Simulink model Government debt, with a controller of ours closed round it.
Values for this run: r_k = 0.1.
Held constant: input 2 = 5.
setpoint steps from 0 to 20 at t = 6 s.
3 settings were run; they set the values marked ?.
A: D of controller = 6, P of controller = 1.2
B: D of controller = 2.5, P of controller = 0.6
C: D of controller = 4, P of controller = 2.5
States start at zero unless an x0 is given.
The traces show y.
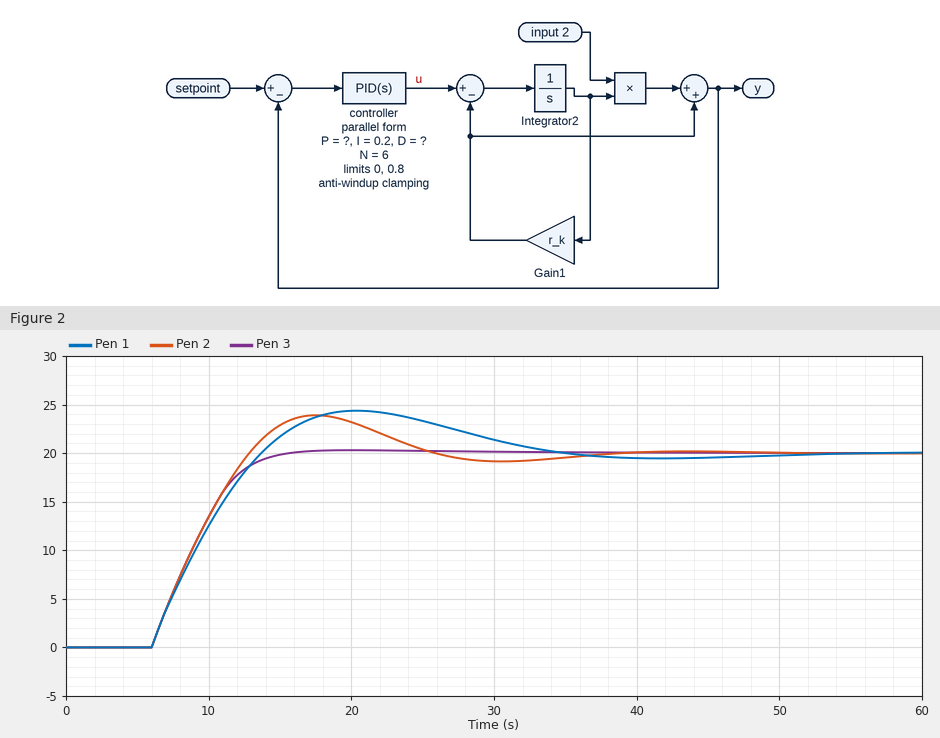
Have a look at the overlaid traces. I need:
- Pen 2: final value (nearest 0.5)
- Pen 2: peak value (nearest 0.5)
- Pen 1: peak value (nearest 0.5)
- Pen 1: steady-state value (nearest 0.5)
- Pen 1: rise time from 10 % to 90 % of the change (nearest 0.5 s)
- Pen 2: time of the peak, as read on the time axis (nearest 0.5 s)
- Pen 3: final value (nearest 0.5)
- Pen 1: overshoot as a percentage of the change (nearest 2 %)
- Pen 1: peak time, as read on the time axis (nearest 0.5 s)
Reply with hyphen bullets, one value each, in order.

- 20.0
- 24.0
- 24.5
- 20.0
- 6.0 s
- 17.5 s
- 20.0
- 22 %
- 20.5 s
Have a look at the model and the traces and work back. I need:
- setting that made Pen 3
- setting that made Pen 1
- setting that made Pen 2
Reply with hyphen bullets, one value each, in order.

- C
- A
- B
